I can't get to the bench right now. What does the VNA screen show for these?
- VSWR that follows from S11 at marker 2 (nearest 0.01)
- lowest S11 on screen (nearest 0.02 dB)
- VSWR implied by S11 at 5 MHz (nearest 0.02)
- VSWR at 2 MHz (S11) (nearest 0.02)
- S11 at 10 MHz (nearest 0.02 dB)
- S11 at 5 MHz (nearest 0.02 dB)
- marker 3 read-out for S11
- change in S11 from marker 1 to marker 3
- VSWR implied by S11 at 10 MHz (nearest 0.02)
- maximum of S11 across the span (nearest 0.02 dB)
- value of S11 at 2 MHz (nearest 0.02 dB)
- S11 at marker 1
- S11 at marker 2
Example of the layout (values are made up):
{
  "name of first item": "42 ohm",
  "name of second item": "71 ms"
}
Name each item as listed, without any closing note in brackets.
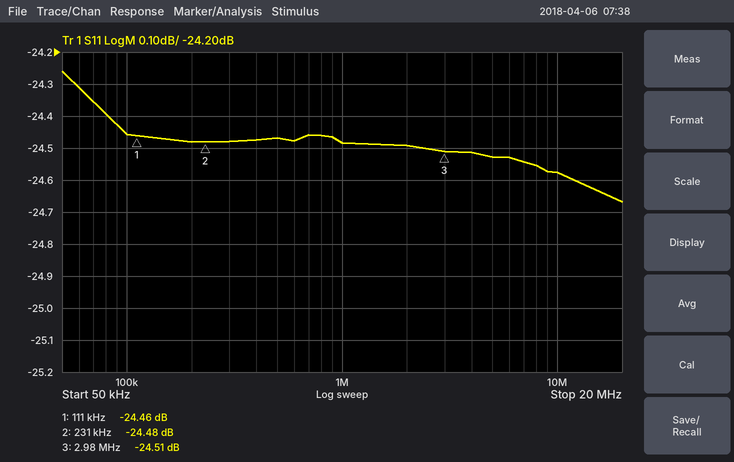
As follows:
{
  "VSWR that follows from S11 at marker 2": "1.13",
  "lowest S11 on screen": "-24.66 dB",
  "VSWR implied by S11 at 5 MHz": "1.12",
  "VSWR at 2 MHz (S11)": "1.12",
  "S11 at 10 MHz": "-24.58 dB",
  "S11 at 5 MHz": "-24.52 dB",
  "marker 3 read-out for S11": "-24.51 dB",
  "change in S11 from marker 1 to marker 3": "-0.05 dB",
  "VSWR implied by S11 at 10 MHz": "1.12",
  "maximum of S11 across the span": "-24.26 dB",
  "value of S11 at 2 MHz": "-24.50 dB",
  "S11 at marker 1": "-24.46 dB",
  "S11 at marker 2": "-24.48 dB"
}
